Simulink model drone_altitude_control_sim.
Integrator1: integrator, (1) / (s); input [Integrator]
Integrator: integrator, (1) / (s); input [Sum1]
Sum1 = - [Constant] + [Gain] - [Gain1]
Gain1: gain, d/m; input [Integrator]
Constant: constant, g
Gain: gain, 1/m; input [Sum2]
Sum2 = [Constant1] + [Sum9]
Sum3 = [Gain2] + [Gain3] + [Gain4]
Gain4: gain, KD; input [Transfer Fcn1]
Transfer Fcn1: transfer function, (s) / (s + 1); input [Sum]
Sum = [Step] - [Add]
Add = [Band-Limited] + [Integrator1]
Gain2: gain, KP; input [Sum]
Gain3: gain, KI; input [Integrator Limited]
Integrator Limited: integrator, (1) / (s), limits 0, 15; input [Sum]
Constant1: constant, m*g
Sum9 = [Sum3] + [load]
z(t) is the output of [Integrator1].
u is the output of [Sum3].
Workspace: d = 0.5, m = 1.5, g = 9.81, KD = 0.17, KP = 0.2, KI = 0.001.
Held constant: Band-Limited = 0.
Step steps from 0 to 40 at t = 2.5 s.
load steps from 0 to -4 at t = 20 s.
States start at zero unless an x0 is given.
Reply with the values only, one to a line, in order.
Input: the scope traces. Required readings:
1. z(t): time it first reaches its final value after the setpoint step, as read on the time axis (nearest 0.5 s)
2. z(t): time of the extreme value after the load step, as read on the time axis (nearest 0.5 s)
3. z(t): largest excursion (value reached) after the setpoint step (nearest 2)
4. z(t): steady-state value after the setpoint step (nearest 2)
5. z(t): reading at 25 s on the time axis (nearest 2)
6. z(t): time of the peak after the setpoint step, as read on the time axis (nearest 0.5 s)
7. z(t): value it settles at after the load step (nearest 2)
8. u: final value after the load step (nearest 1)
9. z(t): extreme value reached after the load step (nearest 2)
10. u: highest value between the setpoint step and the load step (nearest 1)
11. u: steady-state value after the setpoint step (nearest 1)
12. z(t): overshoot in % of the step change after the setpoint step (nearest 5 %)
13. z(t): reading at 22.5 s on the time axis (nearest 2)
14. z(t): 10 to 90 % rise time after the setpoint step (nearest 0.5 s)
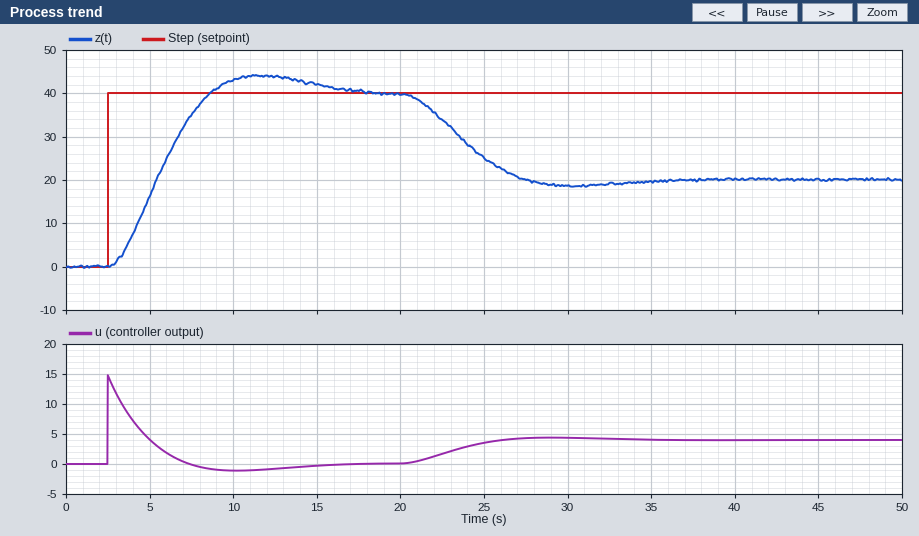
8.5 s
30.5 s
44
40
26
11.5 s
20
4
18
15
0
10 %
34
4.0 s
